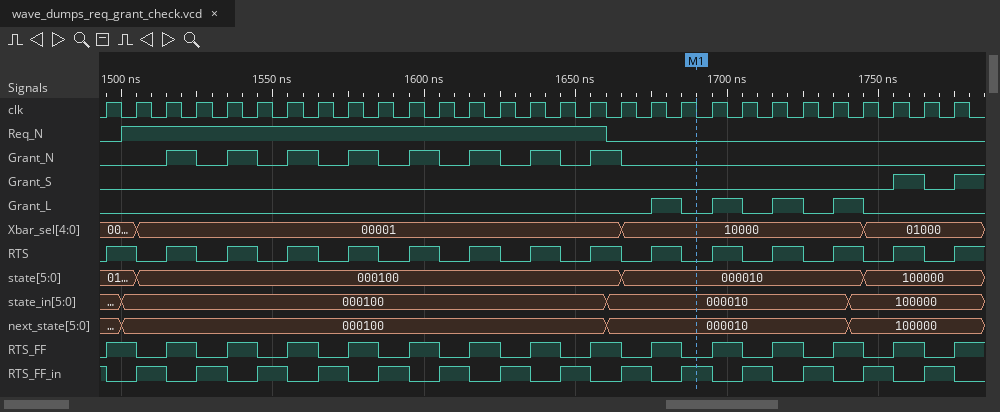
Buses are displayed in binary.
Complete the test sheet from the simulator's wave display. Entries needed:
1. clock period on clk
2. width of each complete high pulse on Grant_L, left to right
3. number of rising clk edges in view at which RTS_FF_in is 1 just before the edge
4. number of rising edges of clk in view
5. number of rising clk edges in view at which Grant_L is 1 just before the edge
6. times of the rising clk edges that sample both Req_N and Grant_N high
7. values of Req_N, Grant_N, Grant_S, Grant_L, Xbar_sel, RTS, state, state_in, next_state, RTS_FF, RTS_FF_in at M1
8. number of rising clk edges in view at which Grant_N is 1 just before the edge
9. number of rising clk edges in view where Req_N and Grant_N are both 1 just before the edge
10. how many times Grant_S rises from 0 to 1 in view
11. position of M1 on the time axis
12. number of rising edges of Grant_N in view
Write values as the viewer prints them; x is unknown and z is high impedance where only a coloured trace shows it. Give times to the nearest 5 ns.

10 ns
10 ns, 10 ns, 10 ns, 10 ns
15
29
4
1525 ns, 1545 ns, 1565 ns, 1585 ns, 1605 ns, 1625 ns, 1645 ns
Req_N=0, Grant_N=0, Grant_S=0, Grant_L=0, Xbar_sel=10000, RTS=0, state=000010, state_in=000010, next_state=000010, RTS_FF=0, RTS_FF_in=1
8
7
2
1690 ns
8
